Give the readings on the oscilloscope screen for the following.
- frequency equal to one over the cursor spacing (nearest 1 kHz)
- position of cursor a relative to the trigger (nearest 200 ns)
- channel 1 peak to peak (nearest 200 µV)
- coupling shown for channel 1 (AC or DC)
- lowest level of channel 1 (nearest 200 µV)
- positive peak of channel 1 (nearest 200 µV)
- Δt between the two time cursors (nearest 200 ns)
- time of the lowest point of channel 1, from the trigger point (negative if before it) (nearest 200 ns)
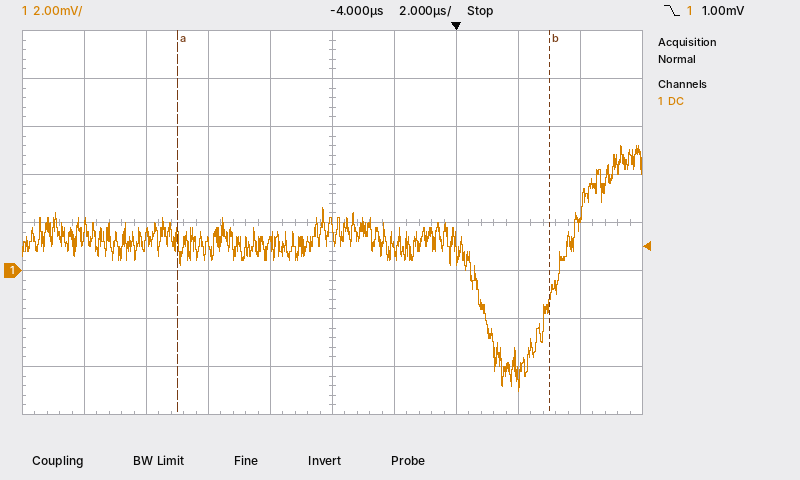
83 kHz
-9.0 µs
10.2 mV
DC
-5.0 mV
5.2 mV
12.0 µs
+2.0 µs
